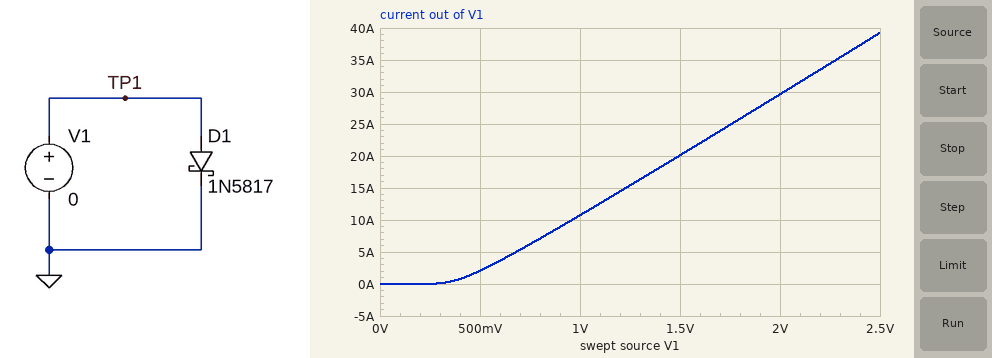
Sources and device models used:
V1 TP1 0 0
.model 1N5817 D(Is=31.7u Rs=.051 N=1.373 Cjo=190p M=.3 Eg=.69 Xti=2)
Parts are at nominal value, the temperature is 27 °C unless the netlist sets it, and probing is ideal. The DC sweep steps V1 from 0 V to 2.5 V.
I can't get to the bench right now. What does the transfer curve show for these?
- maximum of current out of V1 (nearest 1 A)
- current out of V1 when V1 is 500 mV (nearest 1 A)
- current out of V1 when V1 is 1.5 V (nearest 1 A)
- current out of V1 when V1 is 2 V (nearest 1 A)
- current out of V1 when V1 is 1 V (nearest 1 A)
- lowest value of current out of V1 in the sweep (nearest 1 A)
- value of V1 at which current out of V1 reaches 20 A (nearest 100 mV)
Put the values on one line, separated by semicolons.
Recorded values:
39 A; 2 A; 20 A; 30 A; 11 A; 0 A; 1.5 V
